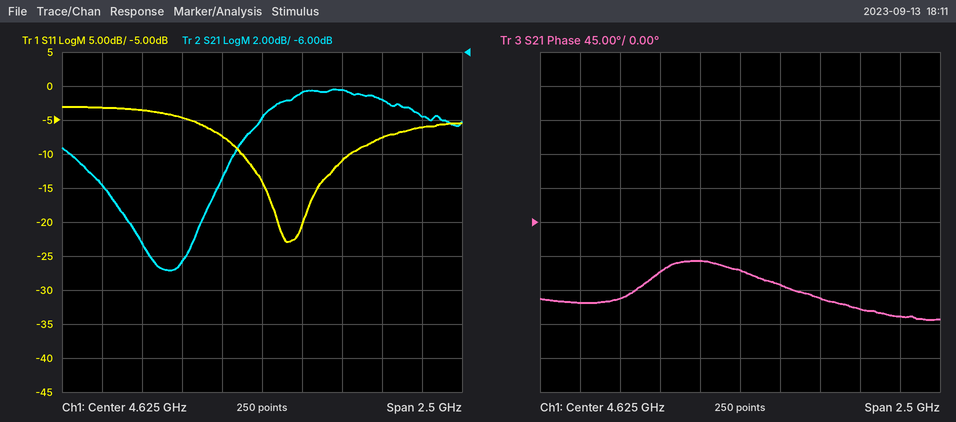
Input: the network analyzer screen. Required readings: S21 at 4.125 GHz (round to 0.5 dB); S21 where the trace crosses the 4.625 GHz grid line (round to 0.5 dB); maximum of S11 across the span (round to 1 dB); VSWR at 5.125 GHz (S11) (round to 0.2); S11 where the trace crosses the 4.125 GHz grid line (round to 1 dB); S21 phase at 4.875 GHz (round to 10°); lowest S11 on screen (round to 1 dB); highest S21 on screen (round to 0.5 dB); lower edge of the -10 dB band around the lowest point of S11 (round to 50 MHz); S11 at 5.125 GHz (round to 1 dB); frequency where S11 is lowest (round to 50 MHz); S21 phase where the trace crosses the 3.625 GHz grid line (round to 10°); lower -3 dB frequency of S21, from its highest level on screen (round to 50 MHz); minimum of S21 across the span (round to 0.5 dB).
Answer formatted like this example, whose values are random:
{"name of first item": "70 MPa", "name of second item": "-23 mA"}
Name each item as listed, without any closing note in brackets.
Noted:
{"S21 at 4.125 GHz": "-18.5 dB", "S21 where the trace crosses the 4.625 GHz grid line": "-10.0 dB", "maximum of S11 across the span": "-3 dB", "VSWR at 5.125 GHz (S11)": "1.8", "S11 where the trace crosses the 4.125 GHz grid line": "-5 dB", "S21 phase at 4.875 GHz": "-80°", "lowest S11 on screen": "-23 dB", "highest S21 on screen": "-8.0 dB", "lower edge of the -10 dB band around the lowest point of S11": "4.50 GHz", "S11 at 5.125 GHz": "-11 dB", "frequency where S11 is lowest": "4.80 GHz", "S21 phase where the trace crosses the 3.625 GHz grid line": "-110°", "lower -3 dB frequency of S21, from its highest level on screen": "4.50 GHz", "minimum of S21 across the span": "-19.0 dB"}
